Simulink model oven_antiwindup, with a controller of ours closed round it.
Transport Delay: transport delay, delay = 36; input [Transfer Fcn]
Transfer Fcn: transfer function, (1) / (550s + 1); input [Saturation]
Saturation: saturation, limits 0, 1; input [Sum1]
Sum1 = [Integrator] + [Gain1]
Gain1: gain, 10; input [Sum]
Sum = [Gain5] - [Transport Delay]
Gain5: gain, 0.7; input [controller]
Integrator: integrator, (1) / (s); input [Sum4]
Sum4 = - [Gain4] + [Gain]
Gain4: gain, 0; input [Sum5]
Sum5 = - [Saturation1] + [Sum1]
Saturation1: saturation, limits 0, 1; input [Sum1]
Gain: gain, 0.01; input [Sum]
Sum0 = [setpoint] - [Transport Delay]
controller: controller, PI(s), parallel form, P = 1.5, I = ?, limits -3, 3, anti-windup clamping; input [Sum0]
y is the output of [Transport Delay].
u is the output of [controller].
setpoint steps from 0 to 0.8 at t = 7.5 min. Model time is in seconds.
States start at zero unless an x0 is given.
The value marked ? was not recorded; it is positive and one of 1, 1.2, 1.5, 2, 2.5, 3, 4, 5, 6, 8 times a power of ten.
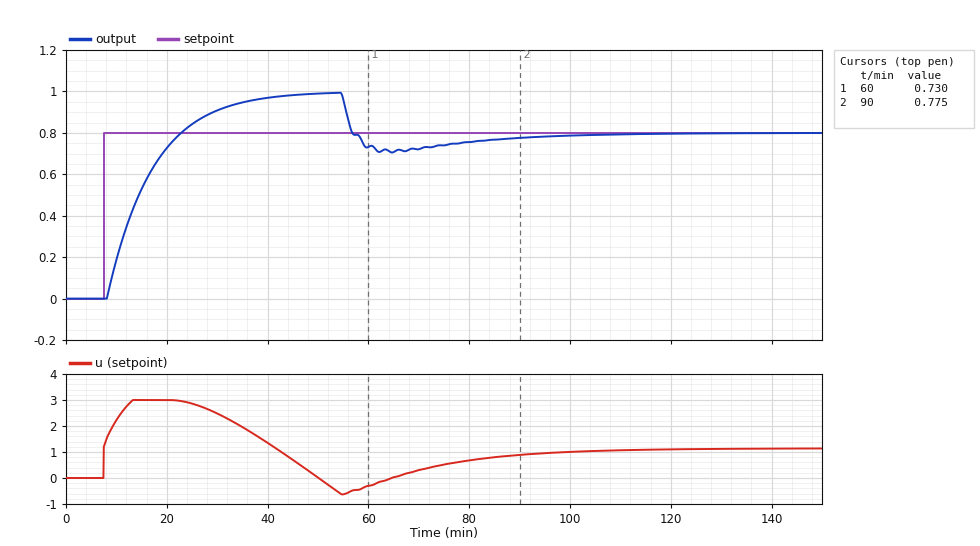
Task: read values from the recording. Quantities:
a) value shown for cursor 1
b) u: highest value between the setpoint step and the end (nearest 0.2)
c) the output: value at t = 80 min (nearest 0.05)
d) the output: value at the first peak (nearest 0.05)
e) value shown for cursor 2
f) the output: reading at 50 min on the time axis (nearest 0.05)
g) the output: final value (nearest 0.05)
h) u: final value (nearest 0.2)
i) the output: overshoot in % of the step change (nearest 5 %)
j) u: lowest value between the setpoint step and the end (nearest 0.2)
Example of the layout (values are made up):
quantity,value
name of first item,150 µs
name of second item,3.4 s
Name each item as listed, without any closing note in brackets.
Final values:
quantity,value
value shown for cursor 1,0.730
u: highest value between the setpoint step and the end,3.0
the output: value at t = 80 min,0.75
the output: value at the first peak,1.00
value shown for cursor 2,0.775
the output: reading at 50 min on the time axis,1.00
the output: final value,0.80
u: final value,1.2
the output: overshoot in % of the step change,25 %
u: lowest value between the setpoint step and the end,-0.6
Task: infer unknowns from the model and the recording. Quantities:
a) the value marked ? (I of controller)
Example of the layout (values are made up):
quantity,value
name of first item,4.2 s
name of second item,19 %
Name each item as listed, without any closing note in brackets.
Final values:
quantity,value
the value marked ?,0.012
